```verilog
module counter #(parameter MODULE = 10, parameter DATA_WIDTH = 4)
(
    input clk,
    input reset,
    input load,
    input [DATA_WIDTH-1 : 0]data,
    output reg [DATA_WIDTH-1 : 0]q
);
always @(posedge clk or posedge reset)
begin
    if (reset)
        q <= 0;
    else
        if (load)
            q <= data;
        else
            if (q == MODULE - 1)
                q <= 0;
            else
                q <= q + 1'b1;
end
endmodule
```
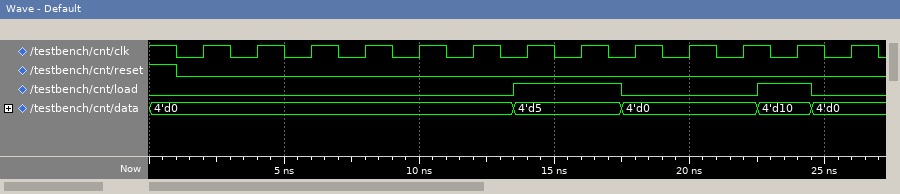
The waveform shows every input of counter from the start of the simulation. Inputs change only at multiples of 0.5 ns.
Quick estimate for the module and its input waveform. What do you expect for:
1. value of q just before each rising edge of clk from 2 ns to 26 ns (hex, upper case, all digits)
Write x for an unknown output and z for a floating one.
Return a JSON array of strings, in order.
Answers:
["0, 1, 2, 3, 4, 5, 6, 5, 5, 6, 7, 8, A"]
